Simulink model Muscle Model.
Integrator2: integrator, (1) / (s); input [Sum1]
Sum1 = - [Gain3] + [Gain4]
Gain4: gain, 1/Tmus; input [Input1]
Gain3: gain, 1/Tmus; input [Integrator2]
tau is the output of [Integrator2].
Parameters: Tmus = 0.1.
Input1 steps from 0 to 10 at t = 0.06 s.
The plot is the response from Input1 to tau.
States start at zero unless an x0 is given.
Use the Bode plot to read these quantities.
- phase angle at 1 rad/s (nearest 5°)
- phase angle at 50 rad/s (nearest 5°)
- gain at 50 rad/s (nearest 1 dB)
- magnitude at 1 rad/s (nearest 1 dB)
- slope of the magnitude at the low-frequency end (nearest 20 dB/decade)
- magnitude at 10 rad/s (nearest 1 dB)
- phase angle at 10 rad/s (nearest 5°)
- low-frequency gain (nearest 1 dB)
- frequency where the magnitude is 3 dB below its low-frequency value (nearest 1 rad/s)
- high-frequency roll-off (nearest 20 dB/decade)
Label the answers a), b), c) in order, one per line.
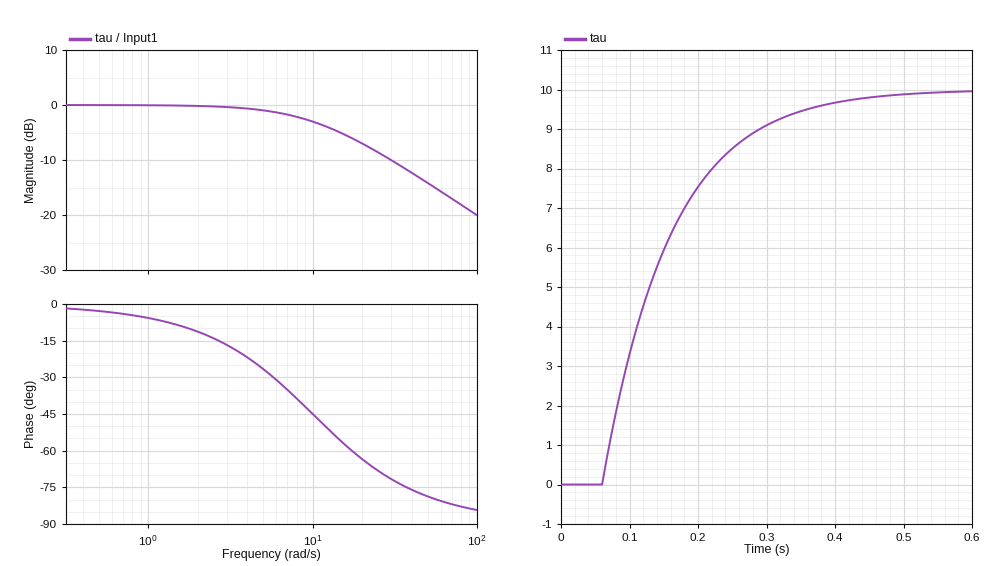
a) -5°
b) -80°
c) -14 dB
d) 0 dB
e) 0 dB/decade
f) -3 dB
g) -45°
h) 0 dB
i) 10 rad/s
j) -20 dB/decade
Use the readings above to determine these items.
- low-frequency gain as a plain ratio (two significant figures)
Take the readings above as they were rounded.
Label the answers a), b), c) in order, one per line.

a) 1.0
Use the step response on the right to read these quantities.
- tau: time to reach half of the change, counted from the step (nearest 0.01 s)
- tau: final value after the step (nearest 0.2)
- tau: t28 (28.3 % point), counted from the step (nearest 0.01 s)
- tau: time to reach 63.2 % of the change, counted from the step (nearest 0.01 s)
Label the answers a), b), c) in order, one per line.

a) 0.07 s
b) 10.0
c) 0.03 s
d) 0.10 s
